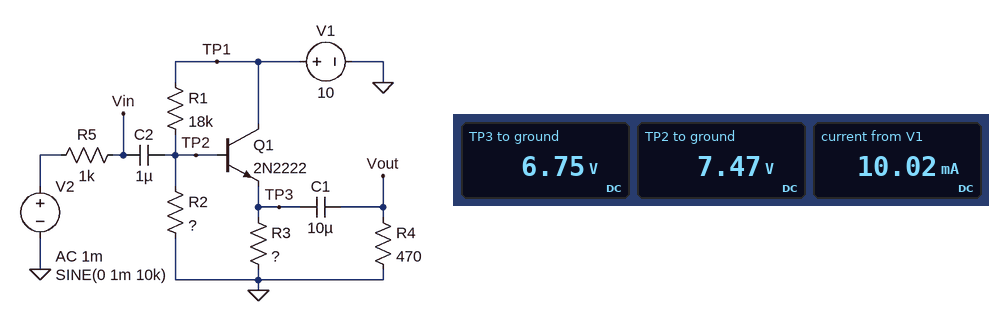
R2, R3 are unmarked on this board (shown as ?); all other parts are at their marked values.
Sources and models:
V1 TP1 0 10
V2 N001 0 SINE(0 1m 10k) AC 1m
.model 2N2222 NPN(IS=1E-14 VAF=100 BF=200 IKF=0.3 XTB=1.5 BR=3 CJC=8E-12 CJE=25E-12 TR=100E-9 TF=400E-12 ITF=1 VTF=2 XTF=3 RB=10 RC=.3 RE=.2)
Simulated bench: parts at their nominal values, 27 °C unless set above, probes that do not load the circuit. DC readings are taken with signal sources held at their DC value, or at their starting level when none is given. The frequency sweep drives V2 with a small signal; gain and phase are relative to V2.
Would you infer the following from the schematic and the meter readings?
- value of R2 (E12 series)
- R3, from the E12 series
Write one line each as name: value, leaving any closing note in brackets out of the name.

value of R2: 82 kΩ
R3, from the E12 series: 680 Ω
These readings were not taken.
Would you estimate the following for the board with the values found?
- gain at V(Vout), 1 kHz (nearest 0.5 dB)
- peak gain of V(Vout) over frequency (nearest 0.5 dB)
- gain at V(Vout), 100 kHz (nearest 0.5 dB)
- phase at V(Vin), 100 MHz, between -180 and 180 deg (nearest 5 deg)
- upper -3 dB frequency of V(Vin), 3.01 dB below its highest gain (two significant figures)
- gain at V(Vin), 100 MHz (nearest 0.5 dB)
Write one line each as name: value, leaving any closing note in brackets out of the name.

gain at V(Vout), 1 kHz: -1.0 dB
peak gain of V(Vout) over frequency: -1.0 dB
gain at V(Vout), 100 kHz: -1.0 dB
phase at V(Vin), 100 MHz, between -180 and 180 deg: -70 deg
upper -3 dB frequency of V(Vin), 3.01 dB below its highest gain: 21 MHz
gain at V(Vin), 100 MHz: -13.0 dB
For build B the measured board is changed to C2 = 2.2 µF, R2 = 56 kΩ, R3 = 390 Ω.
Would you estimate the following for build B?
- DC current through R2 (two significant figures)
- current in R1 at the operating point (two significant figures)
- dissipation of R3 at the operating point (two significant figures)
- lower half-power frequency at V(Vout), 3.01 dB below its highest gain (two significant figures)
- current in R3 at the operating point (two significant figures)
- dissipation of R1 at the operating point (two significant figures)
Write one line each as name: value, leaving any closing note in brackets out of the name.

DC current through R2: 120 µA
current in R1 at the operating point: 190 µA
dissipation of R3 at the operating point: 87 mW
lower half-power frequency at V(Vout), 3.01 dB below its highest gain: 35 Hz
current in R3 at the operating point: 15 mA
dissipation of R1 at the operating point: 660 µW
